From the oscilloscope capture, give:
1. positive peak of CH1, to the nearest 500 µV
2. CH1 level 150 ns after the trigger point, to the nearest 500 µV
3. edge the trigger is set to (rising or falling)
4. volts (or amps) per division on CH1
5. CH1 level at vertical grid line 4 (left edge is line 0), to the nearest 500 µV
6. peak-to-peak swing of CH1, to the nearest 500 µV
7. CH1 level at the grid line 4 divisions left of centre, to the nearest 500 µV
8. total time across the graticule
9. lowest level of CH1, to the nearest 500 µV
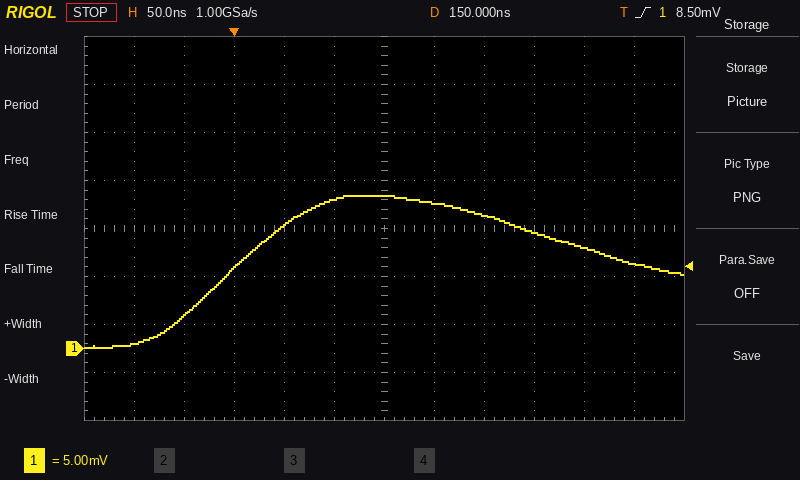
16.0 mV
16.0 mV
rising
5 mV
13.0 mV
16.0 mV
3.5 mV
600 ns
0.0 mV
